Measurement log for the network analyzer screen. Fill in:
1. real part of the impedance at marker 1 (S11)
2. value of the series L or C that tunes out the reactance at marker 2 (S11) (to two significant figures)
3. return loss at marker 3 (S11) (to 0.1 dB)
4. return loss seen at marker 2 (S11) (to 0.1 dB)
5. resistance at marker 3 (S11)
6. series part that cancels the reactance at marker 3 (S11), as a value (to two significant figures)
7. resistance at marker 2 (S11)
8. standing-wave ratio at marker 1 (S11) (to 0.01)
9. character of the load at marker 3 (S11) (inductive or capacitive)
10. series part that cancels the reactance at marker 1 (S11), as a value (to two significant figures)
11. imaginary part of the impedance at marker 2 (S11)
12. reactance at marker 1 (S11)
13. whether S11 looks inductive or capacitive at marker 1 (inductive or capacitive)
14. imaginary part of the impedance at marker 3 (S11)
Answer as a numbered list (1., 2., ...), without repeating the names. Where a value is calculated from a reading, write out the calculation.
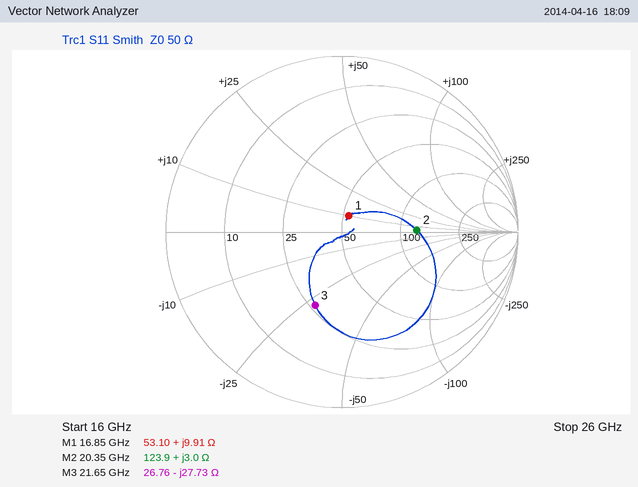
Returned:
1. 53.10 Ω
2. C = 1/(2π × 20.35 GHz × 3 Ω) ≈ 2.6 pF
3. 7.1 dB
4. 7.4 dB
5. 26.76 Ω
6. L = 27.73 Ω/(2π × 21.65 GHz) ≈ 204 pH, so 200 pH to two significant figures
7. 123.9 Ω
8. 1.22
9. capacitive
10. C = 1/(2π × 16.85 GHz × 9.91 Ω) ≈ 953 fF, so 950 fF to two significant figures
11. +3.0 Ω
12. +9.91 Ω
13. inductive
14. -27.73 Ω
